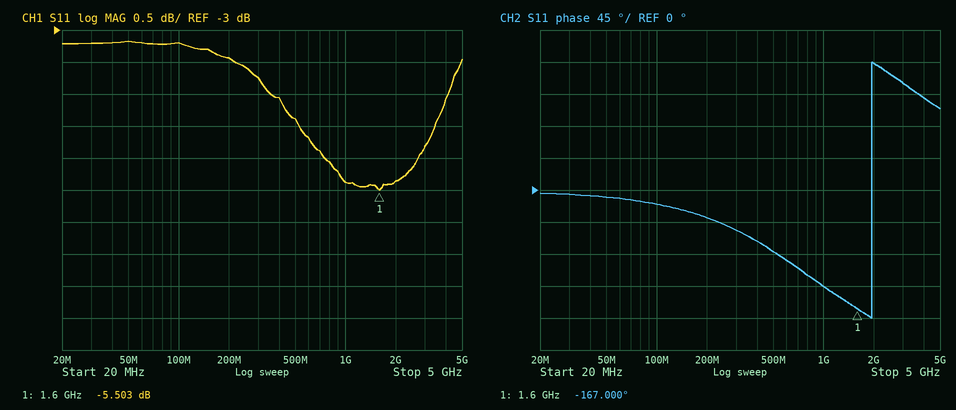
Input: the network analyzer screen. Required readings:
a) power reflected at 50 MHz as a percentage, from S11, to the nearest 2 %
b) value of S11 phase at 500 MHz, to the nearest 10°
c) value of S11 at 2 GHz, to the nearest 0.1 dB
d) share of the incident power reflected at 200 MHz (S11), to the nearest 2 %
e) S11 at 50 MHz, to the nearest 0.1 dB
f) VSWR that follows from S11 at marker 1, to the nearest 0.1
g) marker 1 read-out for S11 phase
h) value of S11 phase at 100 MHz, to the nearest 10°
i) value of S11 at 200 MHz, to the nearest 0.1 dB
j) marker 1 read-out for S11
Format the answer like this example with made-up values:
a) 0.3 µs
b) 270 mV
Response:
a) 48 %
b) -90°
c) -5.4 dB
d) 46 %
e) -3.2 dB
f) 3.3
g) -167.000°
h) -20°
i) -3.4 dB
j) -5.503 dB
